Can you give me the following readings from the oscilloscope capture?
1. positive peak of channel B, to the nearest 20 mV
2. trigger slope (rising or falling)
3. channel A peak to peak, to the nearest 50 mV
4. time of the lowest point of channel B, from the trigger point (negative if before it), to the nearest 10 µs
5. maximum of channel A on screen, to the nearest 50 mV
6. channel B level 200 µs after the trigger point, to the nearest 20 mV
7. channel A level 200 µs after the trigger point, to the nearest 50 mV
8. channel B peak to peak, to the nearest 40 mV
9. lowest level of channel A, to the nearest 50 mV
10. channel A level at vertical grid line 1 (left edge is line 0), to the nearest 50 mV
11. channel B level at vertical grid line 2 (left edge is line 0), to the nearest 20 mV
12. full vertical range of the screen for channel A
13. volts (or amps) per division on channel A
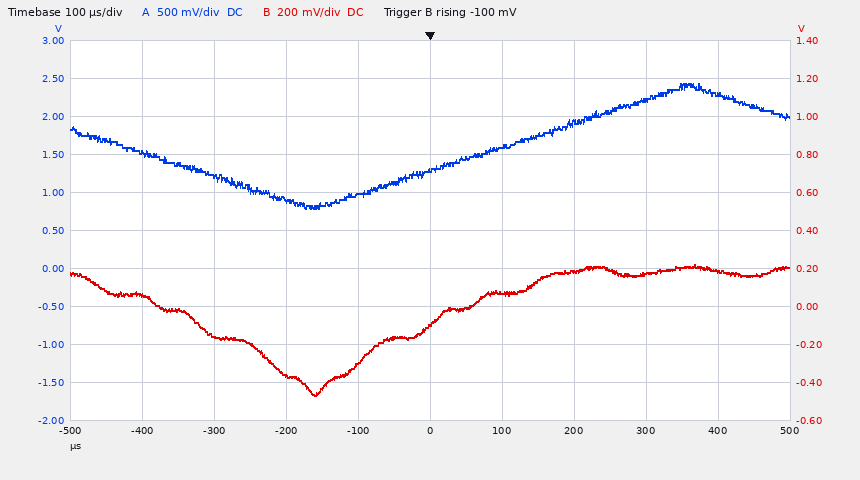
220 mV
rising
1.65 V
-160 µs
2.45 V
180 mV
1.90 V
680 mV
800 mV
1.50 V
-160 mV
5 V
500 mV
